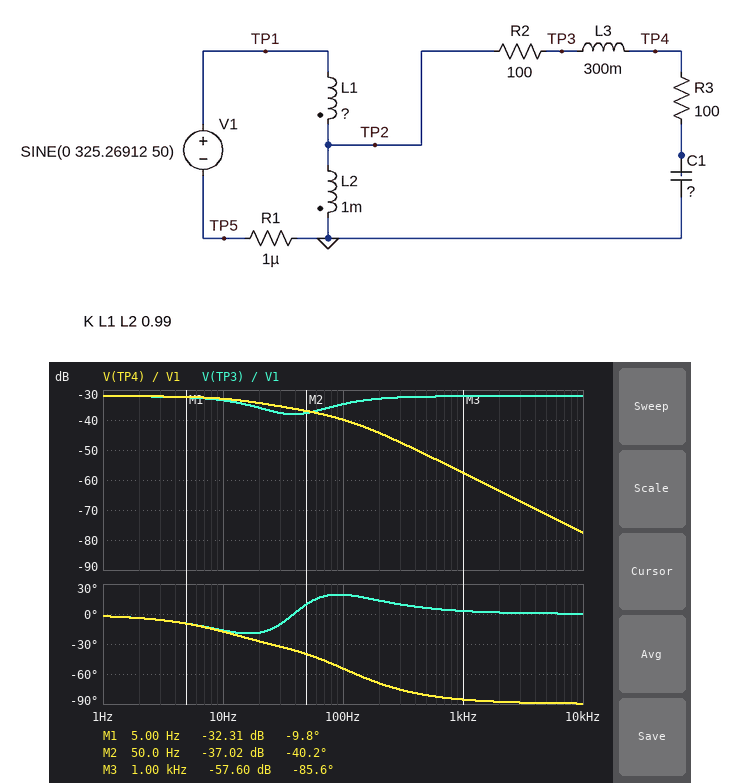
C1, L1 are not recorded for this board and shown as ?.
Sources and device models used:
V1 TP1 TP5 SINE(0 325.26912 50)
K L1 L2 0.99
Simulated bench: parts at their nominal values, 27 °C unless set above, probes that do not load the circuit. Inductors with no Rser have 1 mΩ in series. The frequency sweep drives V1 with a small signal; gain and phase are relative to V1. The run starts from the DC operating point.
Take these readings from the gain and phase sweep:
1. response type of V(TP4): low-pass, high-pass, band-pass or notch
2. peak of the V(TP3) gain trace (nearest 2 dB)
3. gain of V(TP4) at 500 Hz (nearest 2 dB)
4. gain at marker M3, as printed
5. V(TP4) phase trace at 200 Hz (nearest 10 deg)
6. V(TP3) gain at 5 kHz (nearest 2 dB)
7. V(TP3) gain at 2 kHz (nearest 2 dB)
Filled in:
low-pass
-32 dB
-52 dB
-57.60 dB
-70 deg
-32 dB
-32 dB
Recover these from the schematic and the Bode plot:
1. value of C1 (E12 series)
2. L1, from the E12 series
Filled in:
56 µF
1.5 H
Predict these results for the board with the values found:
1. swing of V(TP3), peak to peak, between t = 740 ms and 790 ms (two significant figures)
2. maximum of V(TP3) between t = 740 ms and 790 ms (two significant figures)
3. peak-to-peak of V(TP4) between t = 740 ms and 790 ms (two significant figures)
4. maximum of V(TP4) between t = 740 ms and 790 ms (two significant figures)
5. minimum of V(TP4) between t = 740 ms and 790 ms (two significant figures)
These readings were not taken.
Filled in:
8.5 V
4.3 V
9.2 V
4.6 V
-4.6 V
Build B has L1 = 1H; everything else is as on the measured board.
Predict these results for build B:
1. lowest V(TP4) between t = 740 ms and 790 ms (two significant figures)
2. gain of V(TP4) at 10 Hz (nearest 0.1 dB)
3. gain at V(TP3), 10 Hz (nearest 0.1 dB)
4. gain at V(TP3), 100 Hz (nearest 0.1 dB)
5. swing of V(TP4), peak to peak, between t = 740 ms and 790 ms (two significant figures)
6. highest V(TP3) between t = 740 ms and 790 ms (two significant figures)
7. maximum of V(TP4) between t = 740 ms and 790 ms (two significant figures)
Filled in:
-5.6 V
-31.2 dB
-31.7 dB
-33.0 dB
11 V
5.2 V
5.6 V
